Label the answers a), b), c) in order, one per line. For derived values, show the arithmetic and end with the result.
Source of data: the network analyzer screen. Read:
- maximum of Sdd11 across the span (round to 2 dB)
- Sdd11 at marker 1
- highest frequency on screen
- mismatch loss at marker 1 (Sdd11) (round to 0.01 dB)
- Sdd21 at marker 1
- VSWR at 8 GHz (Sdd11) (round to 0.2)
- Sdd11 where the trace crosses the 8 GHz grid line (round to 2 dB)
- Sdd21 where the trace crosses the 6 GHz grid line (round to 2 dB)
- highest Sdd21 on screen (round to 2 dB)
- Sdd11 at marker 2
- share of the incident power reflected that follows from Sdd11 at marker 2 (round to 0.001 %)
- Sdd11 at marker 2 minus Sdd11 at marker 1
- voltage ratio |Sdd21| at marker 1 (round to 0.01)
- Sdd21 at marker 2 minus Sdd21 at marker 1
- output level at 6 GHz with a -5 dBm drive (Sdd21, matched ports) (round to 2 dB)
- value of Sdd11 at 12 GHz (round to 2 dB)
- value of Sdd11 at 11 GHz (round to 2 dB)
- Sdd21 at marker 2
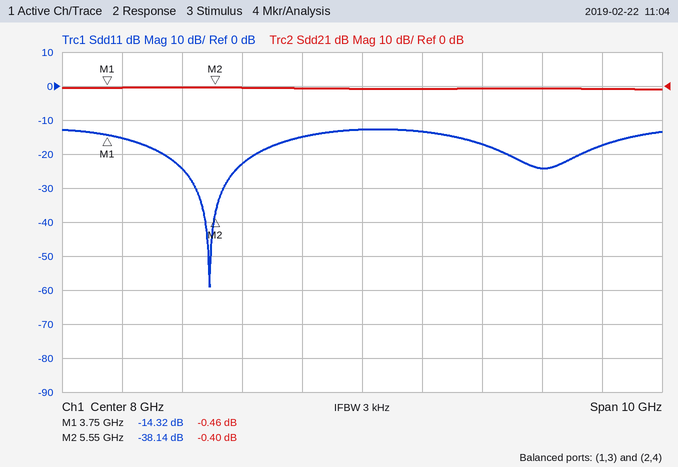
a) -12 dB
b) -14.32 dB
c) 13 GHz
d) −10 log10(1 − 10^(-14.32/10)) ≈ 0.16 dB
e) -0.46 dB
f) |Γ| = 10^(-12/20) = 0.2512; VSWR = (1 + 0.2512)/(1 − 0.2512) ≈ 1.67, so 1.6 to the nearest 0.2
g) -12 dB
h) 0 dB
i) 0 dB
j) -38.14 dB
k) 10^(-38.14/10) ≈ 0.015 %
l) -38.14 − (-14.32) = -23.82 dB
m) 10^(-0.46/20) ≈ 0.95
n) -0.4 − (-0.46) = 0.06 dB
o) -5 dBm + (0 dB) = -6 dBm
p) -18 dB
q) -24 dB
r) -0.40 dB
